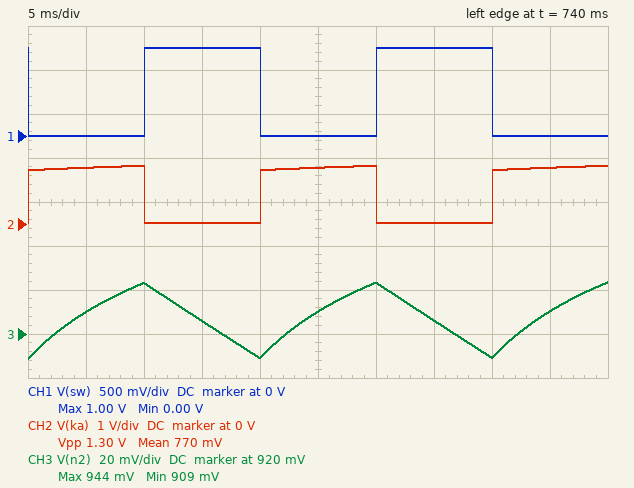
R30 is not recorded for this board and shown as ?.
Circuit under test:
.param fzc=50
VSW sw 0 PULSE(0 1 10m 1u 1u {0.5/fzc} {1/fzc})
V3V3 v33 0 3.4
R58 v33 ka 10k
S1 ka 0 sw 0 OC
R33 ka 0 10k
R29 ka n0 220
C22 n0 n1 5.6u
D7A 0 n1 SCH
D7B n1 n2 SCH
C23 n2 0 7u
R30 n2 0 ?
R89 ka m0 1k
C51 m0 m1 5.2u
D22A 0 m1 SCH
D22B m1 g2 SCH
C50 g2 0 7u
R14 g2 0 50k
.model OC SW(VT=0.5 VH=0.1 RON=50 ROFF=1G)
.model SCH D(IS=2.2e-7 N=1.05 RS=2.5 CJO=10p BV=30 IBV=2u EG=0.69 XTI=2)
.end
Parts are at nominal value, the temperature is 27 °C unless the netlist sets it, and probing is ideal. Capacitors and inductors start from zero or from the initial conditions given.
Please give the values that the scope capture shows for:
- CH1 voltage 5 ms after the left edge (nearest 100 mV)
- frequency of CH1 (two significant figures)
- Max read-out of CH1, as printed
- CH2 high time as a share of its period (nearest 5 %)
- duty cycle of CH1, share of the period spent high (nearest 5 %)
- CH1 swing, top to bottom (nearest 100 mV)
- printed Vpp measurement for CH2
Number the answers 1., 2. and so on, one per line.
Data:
1. 0 V
2. 50 Hz
3. 1.00 V
4. 50 %
5. 50 %
6. 1.0 V
7. 1.30 V
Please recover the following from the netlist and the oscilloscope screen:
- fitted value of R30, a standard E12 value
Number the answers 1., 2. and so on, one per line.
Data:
1. 39 kΩ
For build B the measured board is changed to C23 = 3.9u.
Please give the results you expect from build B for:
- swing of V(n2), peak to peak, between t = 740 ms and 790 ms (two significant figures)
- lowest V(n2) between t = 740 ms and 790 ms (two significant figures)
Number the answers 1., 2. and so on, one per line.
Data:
1. 61 mV
2. 890 mV
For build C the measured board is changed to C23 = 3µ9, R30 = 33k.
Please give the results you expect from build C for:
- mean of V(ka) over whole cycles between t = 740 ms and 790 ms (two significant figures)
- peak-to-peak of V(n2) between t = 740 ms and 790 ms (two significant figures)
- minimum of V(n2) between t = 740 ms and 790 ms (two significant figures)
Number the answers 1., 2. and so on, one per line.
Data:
1. 640 mV
2. 69 mV
3. 850 mV
